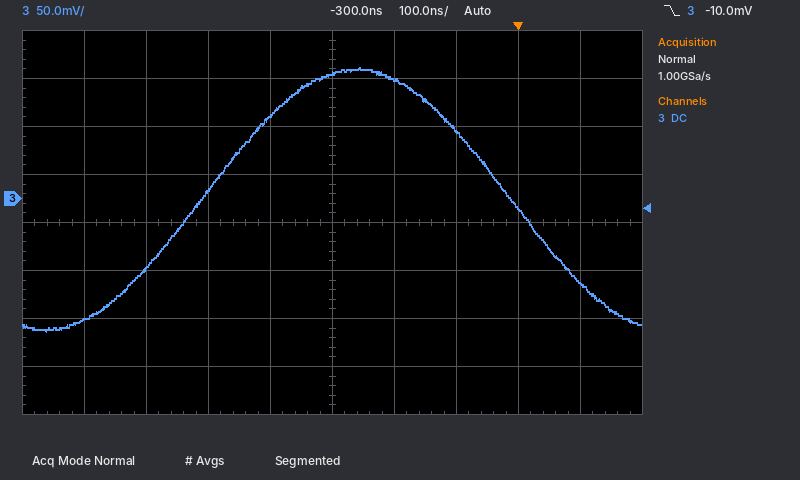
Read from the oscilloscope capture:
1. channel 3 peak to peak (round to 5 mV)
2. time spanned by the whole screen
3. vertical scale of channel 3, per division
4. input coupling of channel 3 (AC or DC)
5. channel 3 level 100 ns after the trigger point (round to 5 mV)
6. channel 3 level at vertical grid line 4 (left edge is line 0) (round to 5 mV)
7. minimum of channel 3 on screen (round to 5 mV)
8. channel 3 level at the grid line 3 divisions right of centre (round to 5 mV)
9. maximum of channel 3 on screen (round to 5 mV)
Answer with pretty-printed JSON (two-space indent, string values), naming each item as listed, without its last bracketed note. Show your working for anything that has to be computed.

{
  "channel 3 peak to peak": "135 mV − (-140 mV) = 275 mV",
  "time spanned by the whole screen": "1 µs",
  "vertical scale of channel 3, per division": "50 mV",
  "input coupling of channel 3": "DC",
  "channel 3 level 100 ns after the trigger point": "-90 mV",
  "channel 3 level at vertical grid line 4 (left edge is line 0)": "85 mV",
  "minimum of channel 3 on screen": "-140 mV",
  "channel 3 level at the grid line 3 divisions right of centre": "-10 mV",
  "maximum of channel 3 on screen": "135 mV"
}
